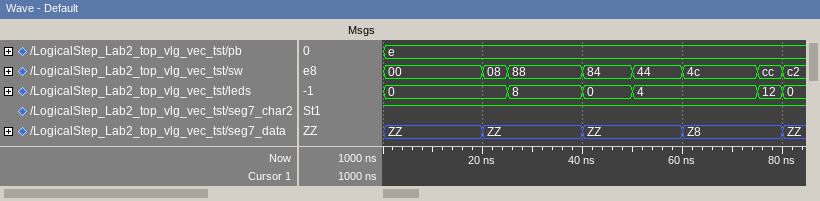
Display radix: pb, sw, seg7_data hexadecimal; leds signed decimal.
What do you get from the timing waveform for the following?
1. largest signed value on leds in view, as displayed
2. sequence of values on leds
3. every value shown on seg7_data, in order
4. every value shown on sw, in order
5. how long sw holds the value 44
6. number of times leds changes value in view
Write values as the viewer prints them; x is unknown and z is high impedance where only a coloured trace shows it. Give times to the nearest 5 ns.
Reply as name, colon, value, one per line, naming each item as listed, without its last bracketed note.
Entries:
largest signed value on leds in view, as displayed: 12
sequence of values on leds: 0, 8, 0, 4, 12, 0
every value shown on seg7_data, in order: ZZ, ZZ, ZZ, Z8, ZZ
every value shown on sw, in order: 00, 08, 88, 84, 44, 4c, cc, c2
how long sw holds the value 44: 10 ns
number of times leds changes value in view: 5
